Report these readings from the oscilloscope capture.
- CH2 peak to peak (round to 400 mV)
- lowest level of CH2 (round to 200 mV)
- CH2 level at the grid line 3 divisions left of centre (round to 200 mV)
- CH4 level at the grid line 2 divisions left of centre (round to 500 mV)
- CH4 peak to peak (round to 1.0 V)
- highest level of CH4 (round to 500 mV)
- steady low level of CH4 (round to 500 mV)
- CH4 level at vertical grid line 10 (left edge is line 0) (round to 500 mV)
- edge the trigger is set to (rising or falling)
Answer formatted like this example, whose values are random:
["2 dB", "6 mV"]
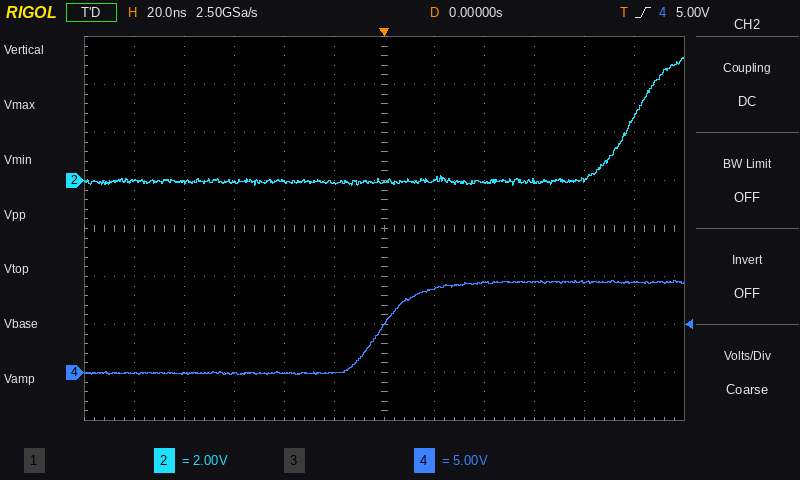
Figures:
["5.2 V", "-200 mV", "0.0 V", "0.0 V", "10.0 V", "9.5 V", "0.0 V", "9.5 V", "rising"]
